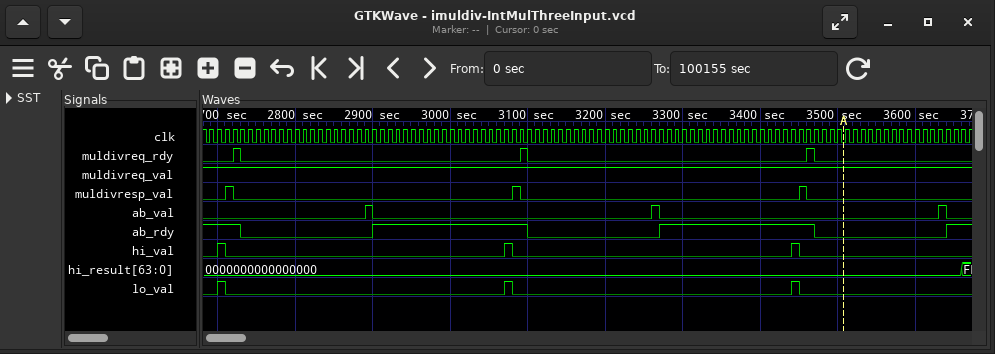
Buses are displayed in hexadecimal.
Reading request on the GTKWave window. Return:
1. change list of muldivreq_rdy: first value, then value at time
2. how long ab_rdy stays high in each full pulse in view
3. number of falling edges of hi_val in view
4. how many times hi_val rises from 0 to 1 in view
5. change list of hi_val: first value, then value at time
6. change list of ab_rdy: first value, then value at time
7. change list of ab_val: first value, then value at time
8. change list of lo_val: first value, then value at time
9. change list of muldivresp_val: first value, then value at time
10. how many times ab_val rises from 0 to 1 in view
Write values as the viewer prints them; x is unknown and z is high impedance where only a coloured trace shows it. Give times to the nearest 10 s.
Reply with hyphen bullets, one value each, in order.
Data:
- 0, 1 at 2720 s, 0 at 2730 s, 1 at 3090 s, 0 at 3100 s, 1 at 3460 s, 0 at 3470 s
- 200 s, 200 s
- 3
- 3
- 0, 1 at 2700 s, 0 at 2710 s, 1 at 3070 s, 0 at 3080 s, 1 at 3440 s, 0 at 3450 s
- 1, 0 at 2730 s, 1 at 2900 s, 0 at 3100 s, 1 at 3270 s, 0 at 3470 s, 1 at 3640 s
- 0, 1 at 2890 s, 0 at 2900 s, 1 at 3260 s, 0 at 3270 s, 1 at 3630 s, 0 at 3640 s
- 0, 1 at 2700 s, 0 at 2710 s, 1 at 3070 s, 0 at 3080 s, 1 at 3440 s, 0 at 3450 s
- 0, 1 at 2710 s, 0 at 2720 s, 1 at 3080 s, 0 at 3090 s, 1 at 3450 s, 0 at 3460 s
- 3
